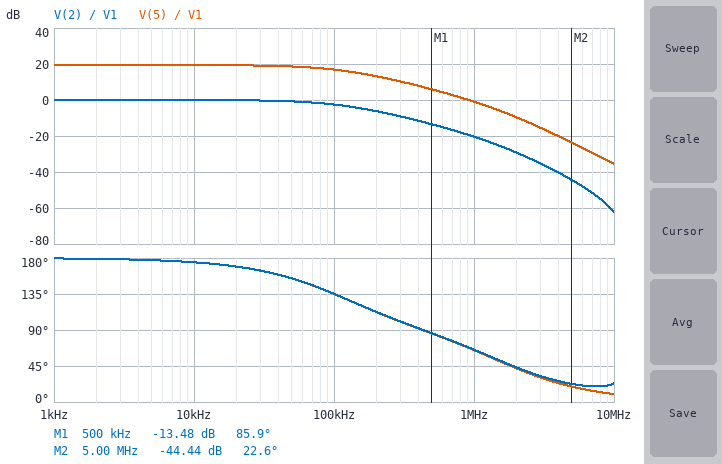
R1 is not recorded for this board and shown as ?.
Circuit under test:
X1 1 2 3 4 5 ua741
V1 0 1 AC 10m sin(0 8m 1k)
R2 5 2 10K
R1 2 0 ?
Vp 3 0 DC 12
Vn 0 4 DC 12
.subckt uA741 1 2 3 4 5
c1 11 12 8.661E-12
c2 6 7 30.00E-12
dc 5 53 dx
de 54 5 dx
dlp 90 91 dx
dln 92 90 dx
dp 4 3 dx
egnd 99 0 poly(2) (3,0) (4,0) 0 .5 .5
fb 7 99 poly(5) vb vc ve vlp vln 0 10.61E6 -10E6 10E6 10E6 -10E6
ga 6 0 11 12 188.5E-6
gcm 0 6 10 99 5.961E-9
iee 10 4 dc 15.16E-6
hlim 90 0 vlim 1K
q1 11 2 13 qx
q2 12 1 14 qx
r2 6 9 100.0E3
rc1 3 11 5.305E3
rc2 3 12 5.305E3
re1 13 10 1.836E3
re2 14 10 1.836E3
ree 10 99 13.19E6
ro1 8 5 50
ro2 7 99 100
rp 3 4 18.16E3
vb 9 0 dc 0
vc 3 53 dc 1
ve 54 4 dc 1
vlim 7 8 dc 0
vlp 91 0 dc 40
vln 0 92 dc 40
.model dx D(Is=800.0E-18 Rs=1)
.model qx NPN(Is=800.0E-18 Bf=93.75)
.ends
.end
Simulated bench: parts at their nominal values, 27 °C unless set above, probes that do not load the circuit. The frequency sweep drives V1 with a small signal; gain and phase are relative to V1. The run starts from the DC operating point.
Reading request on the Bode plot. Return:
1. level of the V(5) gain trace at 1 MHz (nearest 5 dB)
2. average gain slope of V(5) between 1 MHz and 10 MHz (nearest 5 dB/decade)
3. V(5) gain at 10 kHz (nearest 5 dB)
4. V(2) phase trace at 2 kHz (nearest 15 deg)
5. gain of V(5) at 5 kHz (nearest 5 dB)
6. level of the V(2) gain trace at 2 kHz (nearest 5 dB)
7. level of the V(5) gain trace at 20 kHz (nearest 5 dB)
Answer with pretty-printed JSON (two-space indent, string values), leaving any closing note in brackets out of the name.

{
  "level of the V(5) gain trace at 1 MHz": "0 dB",
  "average gain slope of V(5) between 1 MHz and 10 MHz": "-35 dB/decade",
  "V(5) gain at 10 kHz": "20 dB",
  "V(2) phase trace at 2 kHz": "180 deg",
  "gain of V(5) at 5 kHz": "20 dB",
  "level of the V(2) gain trace at 2 kHz": "0 dB",
  "level of the V(5) gain trace at 20 kHz": "20 dB"
}
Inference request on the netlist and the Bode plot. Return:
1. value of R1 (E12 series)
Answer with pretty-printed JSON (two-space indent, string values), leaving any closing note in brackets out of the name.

{
  "value of R1": "1.2 kΩ"
}
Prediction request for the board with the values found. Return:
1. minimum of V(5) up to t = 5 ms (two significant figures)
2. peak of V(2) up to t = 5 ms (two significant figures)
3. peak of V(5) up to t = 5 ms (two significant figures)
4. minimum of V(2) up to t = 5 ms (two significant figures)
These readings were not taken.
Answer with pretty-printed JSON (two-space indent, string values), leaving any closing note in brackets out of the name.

{
  "minimum of V(5) up to t = 5 ms": "-74 mV",
  "peak of V(2) up to t = 5 ms": "8.0 mV",
  "peak of V(5) up to t = 5 ms": "76 mV",
  "minimum of V(2) up to t = 5 ms": "-8.0 mV"
}
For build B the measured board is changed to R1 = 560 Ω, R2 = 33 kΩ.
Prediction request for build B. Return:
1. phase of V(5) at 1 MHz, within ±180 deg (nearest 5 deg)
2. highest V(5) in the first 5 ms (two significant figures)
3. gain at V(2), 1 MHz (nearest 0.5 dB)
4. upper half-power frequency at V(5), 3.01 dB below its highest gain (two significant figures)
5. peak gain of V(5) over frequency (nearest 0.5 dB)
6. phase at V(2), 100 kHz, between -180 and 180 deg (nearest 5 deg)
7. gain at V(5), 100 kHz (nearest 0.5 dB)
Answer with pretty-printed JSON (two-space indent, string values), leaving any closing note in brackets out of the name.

{
  "phase of V(5) at 1 MHz, within ±180 deg": "60 deg",
  "highest V(5) in the first 5 ms": "480 mV",
  "gain at V(2), 1 MHz": "-37.0 dB",
  "upper half-power frequency at V(5), 3.01 dB below its highest gain": "17 kHz",
  "peak gain of V(5) over frequency": "35.5 dB",
  "phase at V(2), 100 kHz, between -180 and 180 deg": "95 deg",
  "gain at V(5), 100 kHz": "20.0 dB"
}
